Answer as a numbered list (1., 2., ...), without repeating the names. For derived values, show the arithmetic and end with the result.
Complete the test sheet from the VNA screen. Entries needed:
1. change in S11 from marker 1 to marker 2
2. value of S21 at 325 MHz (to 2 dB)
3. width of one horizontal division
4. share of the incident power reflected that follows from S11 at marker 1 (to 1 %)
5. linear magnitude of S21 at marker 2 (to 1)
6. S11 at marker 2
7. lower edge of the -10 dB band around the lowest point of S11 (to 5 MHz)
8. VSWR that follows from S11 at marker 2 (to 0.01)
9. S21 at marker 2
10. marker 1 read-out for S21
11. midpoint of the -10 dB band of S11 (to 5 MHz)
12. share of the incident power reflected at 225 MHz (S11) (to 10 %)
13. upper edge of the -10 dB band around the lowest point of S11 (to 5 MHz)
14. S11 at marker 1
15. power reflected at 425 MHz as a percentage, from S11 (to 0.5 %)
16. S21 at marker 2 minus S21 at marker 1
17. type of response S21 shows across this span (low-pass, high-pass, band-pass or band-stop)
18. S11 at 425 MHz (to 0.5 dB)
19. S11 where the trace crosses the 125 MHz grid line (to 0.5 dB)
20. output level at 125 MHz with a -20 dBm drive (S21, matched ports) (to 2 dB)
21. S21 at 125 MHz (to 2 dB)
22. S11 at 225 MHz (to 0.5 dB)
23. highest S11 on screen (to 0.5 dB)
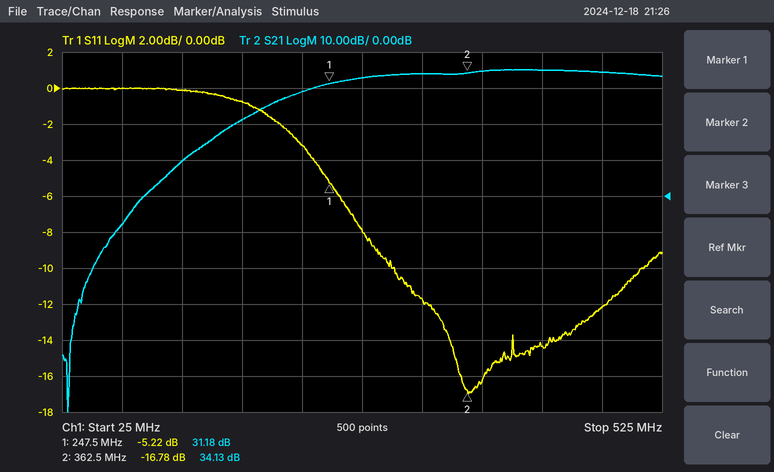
1. -16.78 − (-5.22) = -11.56 dB
2. 34 dB
3. 50 MHz
4. 10^(-5.22/10) ≈ 30 %
5. 10^(34.13/20) ≈ 51
6. -16.78 dB
7. 300 MHz
8. (1 + 0.1449)/(1 − 0.1449) ≈ 1.34
9. 34.13 dB
10. 31.18 dB
11. 405 MHz
12. 10^(-3/10) ≈ 50 %
13. 510 MHz
14. -5.22 dB
15. 10^(-14.5/10) ≈ 3.5 %
16. 34.13 − (31.18) = 2.95 dB
17. high-pass
18. -14.5 dB
19. 0.0 dB
20. -20 dBm + (10 dB) = -10 dBm
21. 10 dB
22. -3.0 dB
23. 0.0 dB
